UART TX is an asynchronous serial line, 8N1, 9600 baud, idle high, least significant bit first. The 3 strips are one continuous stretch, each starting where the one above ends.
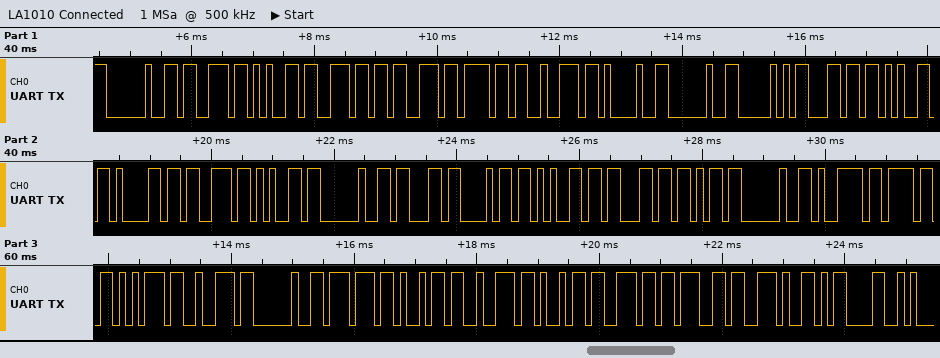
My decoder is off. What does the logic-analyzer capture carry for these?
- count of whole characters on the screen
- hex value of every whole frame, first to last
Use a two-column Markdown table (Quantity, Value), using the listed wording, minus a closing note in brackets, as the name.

| Quantity | Value |
|---|---|
| count of whole characters on the screen | 35 |
| hex value of every whole frame, first to last | 20 73 65 6E 73 6F 72 21 20 50 6C 65 61 73 65 20 63 68 65 63 6B 20 79 6F 75 72 20 77 69 72 69 6E 67 2E 0D |
